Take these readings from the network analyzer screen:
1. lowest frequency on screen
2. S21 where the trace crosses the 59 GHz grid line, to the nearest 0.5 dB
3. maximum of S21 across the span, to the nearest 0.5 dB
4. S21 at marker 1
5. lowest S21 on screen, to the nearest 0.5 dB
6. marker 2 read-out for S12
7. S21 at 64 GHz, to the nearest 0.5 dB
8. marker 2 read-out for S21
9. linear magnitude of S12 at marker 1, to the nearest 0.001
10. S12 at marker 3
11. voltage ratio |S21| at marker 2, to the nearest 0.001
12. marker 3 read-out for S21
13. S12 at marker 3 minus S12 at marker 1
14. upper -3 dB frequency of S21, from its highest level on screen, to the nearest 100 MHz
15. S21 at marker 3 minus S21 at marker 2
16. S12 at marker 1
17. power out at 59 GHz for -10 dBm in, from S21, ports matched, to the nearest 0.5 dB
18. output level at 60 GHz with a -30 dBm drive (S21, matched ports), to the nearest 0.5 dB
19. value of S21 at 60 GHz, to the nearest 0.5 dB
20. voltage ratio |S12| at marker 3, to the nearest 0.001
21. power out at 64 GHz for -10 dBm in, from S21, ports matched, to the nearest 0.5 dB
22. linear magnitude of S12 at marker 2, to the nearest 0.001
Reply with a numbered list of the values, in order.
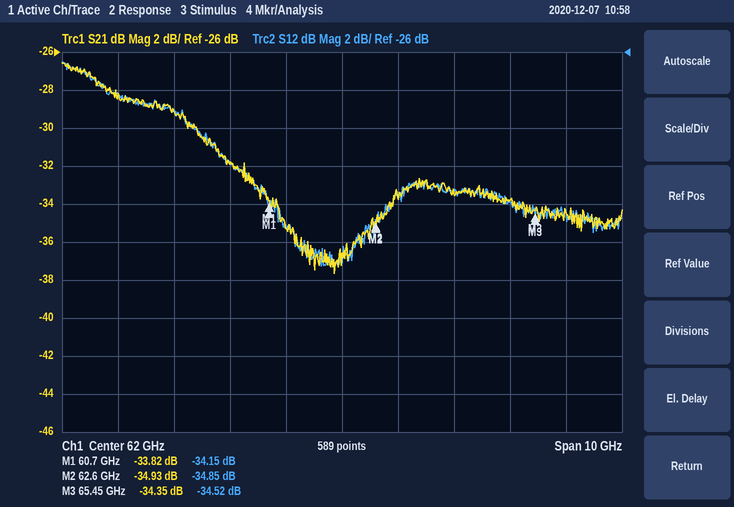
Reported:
1. 57 GHz
2. -29.0 dB
3. -26.5 dB
4. -33.82 dB
5. -37.5 dB
6. -34.85 dB
7. -33.5 dB
8. -34.93 dB
9. 0.020
10. -34.52 dB
11. 0.018
12. -34.35 dB
13. -0.37 dB
14. 59.2 GHz
15. 0.58 dB
16. -34.15 dB
17. -39.0 dBm
18. -62.0 dBm
19. -32.0 dB
20. 0.019
21. -43.5 dBm
22. 0.018
